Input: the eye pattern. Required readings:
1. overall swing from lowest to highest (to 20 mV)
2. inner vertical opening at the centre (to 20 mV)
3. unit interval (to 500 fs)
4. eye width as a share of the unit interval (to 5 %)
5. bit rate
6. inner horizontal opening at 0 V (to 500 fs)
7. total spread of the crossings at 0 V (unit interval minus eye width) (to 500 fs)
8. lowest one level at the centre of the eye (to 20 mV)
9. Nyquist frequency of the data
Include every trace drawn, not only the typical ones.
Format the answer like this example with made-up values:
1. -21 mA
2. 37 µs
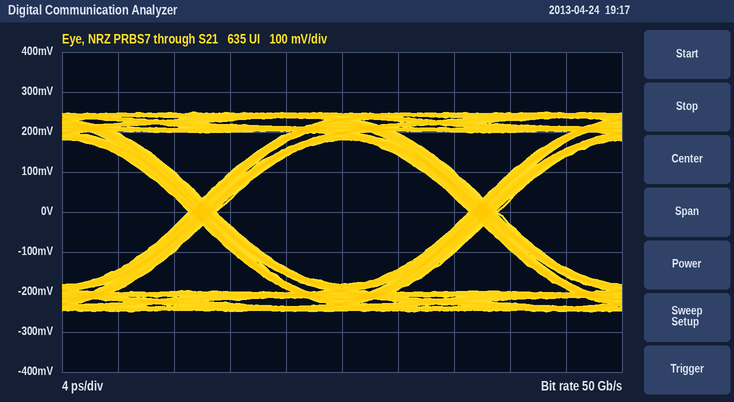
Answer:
1. 500 mV
2. 360 mV
3. 20.0 ps
4. 90 %
5. 50 Gb/s
6. 18.0 ps
7. 2.0 ps
8. 180 mV
9. 25 GHz
